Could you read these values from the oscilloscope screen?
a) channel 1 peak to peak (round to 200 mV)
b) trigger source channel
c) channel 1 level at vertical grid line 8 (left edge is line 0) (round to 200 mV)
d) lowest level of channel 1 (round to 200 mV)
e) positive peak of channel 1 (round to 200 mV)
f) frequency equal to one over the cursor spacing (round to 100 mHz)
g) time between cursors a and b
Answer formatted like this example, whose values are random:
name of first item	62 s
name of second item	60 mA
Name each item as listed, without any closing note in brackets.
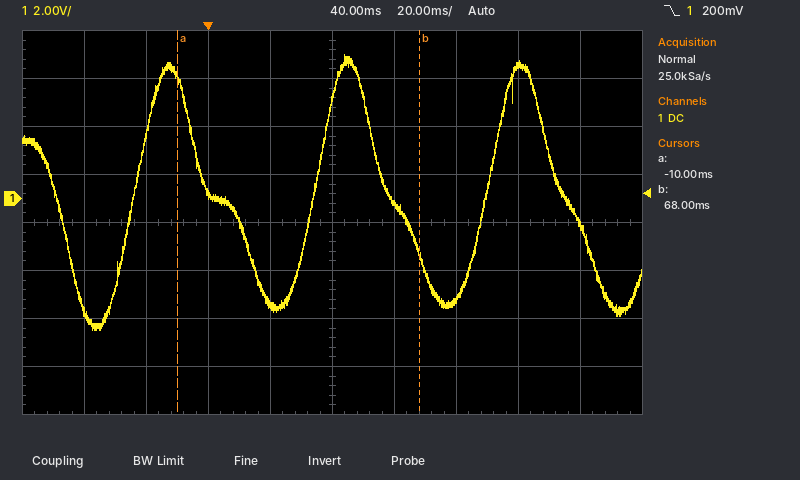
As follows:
channel 1 peak to peak	11.4 V
trigger source channel	channel 1
channel 1 level at vertical grid line 8 (left edge is line 0)	5.6 V
lowest level of channel 1	-5.4 V
positive peak of channel 1	6.0 V
frequency equal to one over the cursor spacing	12.8 Hz
time between cursors a and b	78 ms
